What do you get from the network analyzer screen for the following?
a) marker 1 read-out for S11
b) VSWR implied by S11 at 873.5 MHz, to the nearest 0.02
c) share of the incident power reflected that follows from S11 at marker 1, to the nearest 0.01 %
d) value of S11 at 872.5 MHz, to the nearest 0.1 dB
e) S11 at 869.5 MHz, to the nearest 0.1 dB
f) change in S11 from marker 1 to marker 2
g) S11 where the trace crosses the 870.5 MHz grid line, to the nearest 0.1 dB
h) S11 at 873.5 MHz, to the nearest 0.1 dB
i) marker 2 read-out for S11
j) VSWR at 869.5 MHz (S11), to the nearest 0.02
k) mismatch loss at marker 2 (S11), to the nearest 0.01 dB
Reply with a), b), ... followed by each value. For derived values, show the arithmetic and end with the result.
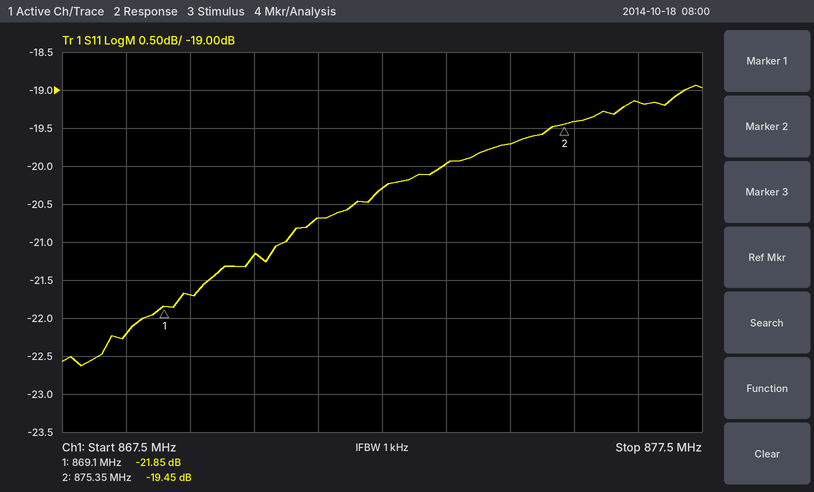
a) -21.85 dB
b) |Γ| = 10^(-20/20) = 0.1000; VSWR = (1 + 0.1000)/(1 − 0.1000) ≈ 1.22
c) 10^(-21.85/10) ≈ 0.65 %
d) -20.3 dB
e) -21.7 dB
f) -19.45 − (-21.85) = 2.40 dB
g) -21.2 dB
h) -20.0 dB
i) -19.45 dB
j) |Γ| = 10^(-21.7/20) = 0.0822; VSWR = (1 + 0.0822)/(1 − 0.0822) ≈ 1.18
k) −10 log10(1 − 10^(-19.45/10)) ≈ 0.05 dB
